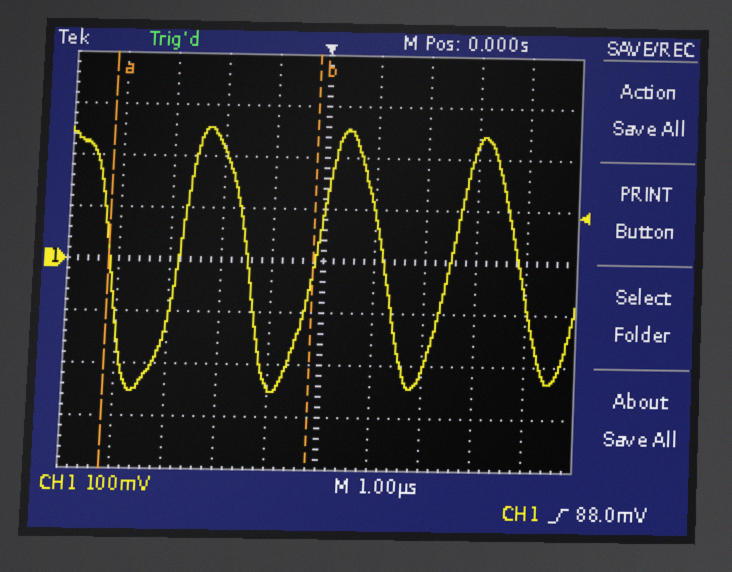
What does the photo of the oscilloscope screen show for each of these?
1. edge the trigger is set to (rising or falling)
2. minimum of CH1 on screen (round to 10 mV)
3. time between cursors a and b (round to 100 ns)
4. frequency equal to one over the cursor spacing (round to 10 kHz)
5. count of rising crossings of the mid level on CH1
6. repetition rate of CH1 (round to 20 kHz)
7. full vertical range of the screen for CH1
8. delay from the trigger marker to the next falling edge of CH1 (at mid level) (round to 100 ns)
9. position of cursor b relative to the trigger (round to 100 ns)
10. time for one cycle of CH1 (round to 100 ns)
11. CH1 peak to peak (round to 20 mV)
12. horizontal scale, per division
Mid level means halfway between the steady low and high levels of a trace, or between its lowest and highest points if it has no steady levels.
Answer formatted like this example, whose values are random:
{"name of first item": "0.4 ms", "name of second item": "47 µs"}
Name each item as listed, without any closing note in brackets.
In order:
{"edge the trigger is set to": "rising", "minimum of CH1 on screen": "-250 mV", "time between cursors a and b": "4.0 µs", "frequency equal to one over the cursor spacing": "250 kHz", "count of rising crossings of the mid level on CH1": "3", "repetition rate of CH1": "380 kHz", "full vertical range of the screen for CH1": "800 mV", "delay from the trigger marker to the next falling edge of CH1 (at mid level)": "1.2 µs", "position of cursor b relative to the trigger": "-200 ns", "time for one cycle of CH1": "2.7 µs", "CH1 peak to peak": "500 mV", "horizontal scale, per division": "1 µs"}
